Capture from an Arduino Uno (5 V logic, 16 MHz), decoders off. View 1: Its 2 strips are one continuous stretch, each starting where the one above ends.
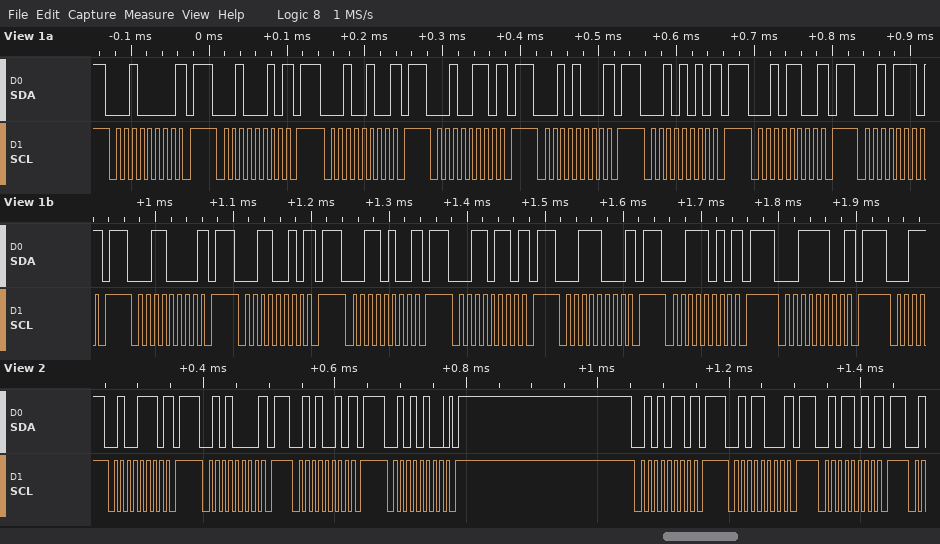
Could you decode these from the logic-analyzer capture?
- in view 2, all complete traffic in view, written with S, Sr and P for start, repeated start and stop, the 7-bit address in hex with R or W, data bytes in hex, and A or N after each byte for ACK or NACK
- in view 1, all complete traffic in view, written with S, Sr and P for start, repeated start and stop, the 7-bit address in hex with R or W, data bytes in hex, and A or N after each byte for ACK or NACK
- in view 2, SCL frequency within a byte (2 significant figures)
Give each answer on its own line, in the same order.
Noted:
S 27W N P S 28W N P S 29W N P S 2AW A P S 2BW N P S 2CW N P S 2DW N P
S 10W N P S 11W N P S 12W N P S 13W N P S 14W N P S 15W N P S 16W N P S 17W N P S 18W N P S 19W N P S 1AW N P S 1BW N P S 1CW N P S 1DW N P S 1EW N P
100 kHz
